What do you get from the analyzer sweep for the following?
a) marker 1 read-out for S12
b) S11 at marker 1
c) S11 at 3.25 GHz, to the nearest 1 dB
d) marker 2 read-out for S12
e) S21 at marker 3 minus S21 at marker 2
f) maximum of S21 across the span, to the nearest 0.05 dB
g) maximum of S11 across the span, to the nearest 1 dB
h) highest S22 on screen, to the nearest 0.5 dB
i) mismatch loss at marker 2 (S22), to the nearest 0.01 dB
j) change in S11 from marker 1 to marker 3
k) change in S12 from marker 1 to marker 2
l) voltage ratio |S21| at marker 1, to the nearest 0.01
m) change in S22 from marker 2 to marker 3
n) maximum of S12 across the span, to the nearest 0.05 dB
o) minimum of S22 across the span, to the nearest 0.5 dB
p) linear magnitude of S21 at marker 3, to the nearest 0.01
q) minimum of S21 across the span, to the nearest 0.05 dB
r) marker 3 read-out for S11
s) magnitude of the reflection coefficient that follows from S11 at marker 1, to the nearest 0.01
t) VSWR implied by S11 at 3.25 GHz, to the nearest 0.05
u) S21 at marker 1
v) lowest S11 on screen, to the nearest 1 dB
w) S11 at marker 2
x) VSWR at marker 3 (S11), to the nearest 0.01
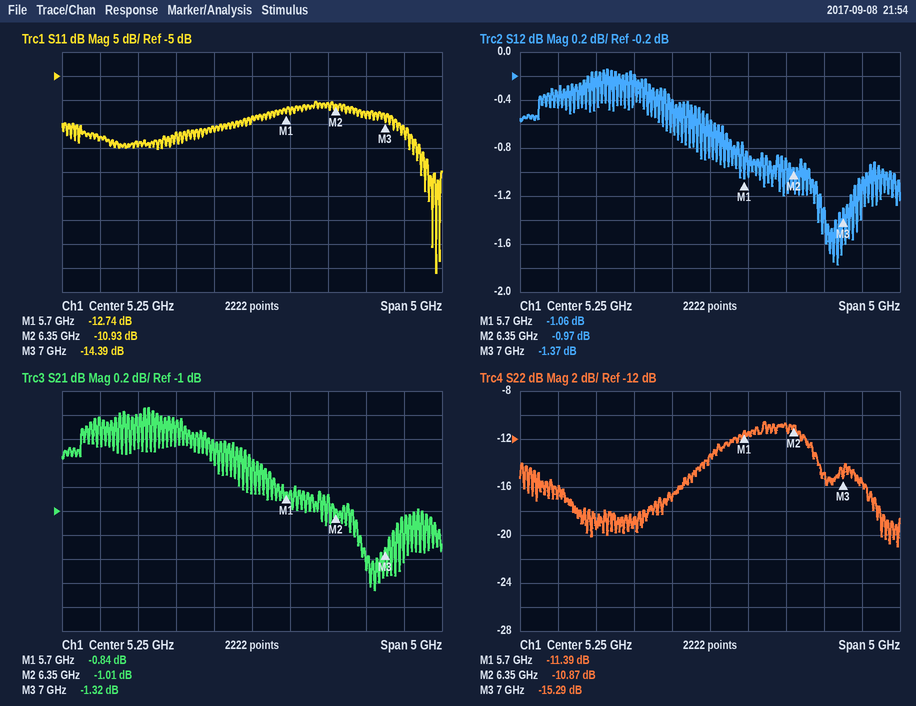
-1.06 dB
-12.74 dB
-18 dB
-0.97 dB
-0.31 dB
-0.15 dB
-10 dB
-10.5 dB
0.37 dB
-1.65 dB
0.09 dB
0.91
-4.42 dB
-0.15 dB
-21.0 dB
0.86
-1.65 dB
-14.39 dB
0.23
1.30
-0.84 dB
-46 dB
-10.93 dB
1.47
